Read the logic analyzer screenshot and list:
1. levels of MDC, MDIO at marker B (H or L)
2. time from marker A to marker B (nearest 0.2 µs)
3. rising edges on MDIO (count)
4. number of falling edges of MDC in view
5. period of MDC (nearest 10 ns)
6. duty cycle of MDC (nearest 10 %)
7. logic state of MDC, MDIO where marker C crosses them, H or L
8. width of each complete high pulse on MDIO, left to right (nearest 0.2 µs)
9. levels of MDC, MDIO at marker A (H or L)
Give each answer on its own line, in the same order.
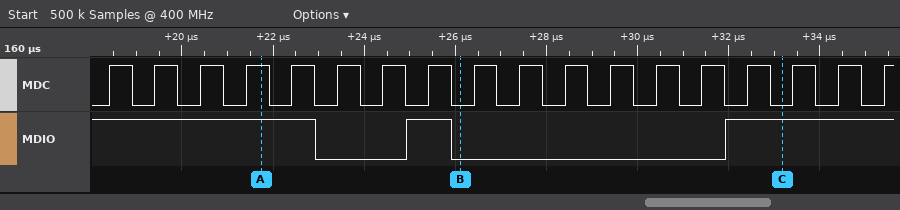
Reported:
MDC=L, MDIO=L
4.4 µs
2
17
1000 ns
50 %
MDC=L, MDIO=H
1 µs
MDC=H, MDIO=H
